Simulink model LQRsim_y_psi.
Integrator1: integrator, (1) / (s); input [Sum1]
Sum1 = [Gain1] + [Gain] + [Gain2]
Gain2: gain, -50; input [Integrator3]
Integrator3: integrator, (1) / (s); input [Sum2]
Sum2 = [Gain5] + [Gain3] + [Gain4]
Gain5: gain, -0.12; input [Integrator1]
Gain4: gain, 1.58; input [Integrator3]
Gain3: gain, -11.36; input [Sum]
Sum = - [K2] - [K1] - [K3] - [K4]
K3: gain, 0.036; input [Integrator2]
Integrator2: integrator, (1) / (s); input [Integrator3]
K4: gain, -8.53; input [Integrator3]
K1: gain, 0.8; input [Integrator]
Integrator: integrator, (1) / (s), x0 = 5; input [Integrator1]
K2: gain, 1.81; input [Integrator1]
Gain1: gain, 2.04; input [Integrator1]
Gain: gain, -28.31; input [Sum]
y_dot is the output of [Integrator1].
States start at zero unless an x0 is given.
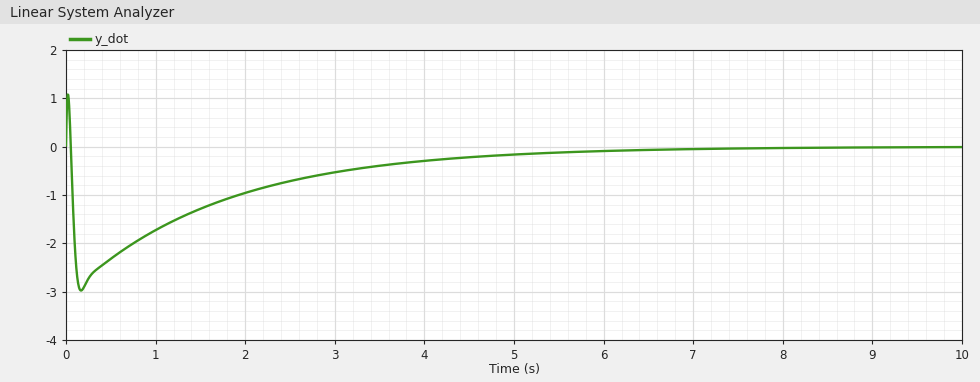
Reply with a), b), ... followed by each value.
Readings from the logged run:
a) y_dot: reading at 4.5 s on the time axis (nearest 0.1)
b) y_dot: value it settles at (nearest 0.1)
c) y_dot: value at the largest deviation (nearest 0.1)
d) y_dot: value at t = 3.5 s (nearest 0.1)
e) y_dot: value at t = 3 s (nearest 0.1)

a) -0.2
b) 0.0
c) -3.0
d) -0.4
e) -0.5
